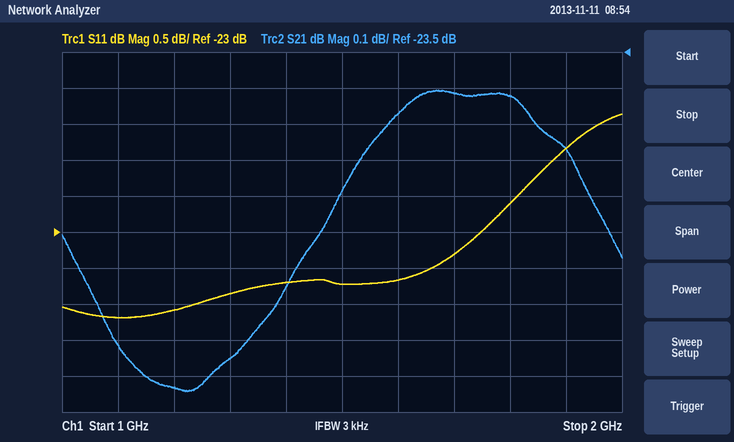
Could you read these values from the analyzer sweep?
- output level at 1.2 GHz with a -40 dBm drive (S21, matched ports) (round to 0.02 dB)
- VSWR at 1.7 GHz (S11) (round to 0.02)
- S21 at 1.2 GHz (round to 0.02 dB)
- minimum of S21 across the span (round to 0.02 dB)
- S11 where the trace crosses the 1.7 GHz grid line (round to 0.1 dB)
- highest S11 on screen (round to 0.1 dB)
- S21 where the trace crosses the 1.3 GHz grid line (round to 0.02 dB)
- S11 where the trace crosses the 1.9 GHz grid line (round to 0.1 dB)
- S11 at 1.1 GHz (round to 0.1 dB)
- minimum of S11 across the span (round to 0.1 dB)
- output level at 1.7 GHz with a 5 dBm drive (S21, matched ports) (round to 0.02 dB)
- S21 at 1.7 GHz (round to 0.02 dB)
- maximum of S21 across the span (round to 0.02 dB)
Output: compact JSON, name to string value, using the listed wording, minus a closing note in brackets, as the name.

{"output level at 1.2 GHz with a -40 dBm drive (S21, matched ports)": "-64.44 dBm", "VSWR at 1.7 GHz (S11)": "1.14", "S21 at 1.2 GHz": "-24.44 dB", "minimum of S21 across the span": "-24.44 dB", "S11 where the trace crosses the 1.7 GHz grid line": "-23.3 dB", "highest S11 on screen": "-21.4 dB", "S21 where the trace crosses the 1.3 GHz grid line": "-24.36 dB", "S11 where the trace crosses the 1.9 GHz grid line": "-21.8 dB", "S11 at 1.1 GHz": "-24.2 dB", "minimum of S11 across the span": "-24.2 dB", "output level at 1.7 GHz with a 5 dBm drive (S21, matched ports)": "-18.62 dBm", "S21 at 1.7 GHz": "-23.62 dB", "maximum of S21 across the span": "-23.60 dB"}
